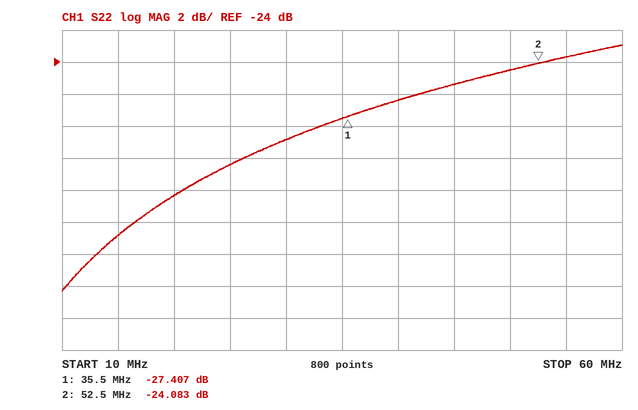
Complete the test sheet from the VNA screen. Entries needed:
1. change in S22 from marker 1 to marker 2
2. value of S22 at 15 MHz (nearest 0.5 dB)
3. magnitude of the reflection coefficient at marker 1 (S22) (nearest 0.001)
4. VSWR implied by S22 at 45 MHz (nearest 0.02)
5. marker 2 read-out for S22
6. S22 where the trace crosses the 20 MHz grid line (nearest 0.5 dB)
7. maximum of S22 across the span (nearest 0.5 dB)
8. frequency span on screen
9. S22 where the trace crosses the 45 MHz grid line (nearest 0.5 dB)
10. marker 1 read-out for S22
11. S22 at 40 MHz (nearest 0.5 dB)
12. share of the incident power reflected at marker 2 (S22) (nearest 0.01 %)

3.324 dB
-35.0 dB
0.043
1.12
-24.083 dB
-32.5 dB
-23.0 dB
50 MHz
-25.5 dB
-27.407 dB
-26.5 dB
0.39 %
